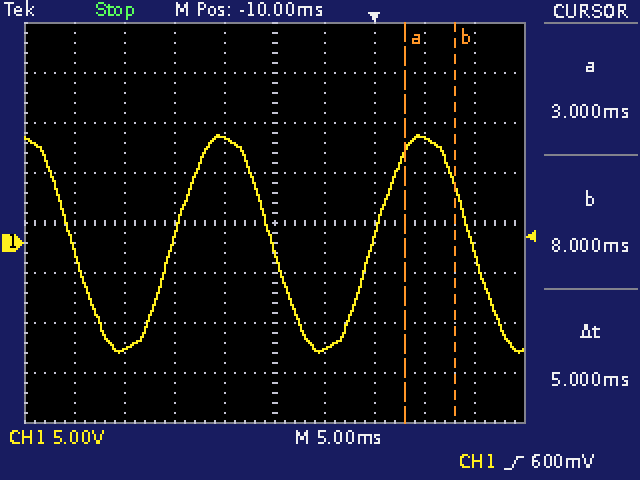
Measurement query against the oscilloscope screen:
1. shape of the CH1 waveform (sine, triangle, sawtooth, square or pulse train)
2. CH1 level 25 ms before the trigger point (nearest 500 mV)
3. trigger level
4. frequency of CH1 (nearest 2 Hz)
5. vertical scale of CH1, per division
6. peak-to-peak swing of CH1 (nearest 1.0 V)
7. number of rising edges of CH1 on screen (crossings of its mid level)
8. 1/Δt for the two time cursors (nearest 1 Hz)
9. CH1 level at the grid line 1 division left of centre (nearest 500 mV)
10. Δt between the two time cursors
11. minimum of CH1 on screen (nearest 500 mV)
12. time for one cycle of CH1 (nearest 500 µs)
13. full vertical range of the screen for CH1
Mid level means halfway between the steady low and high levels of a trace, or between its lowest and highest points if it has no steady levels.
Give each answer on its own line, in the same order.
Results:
sine
-10.5 V
600 mV
50 Hz
5 V
22.0 V
2
200 Hz
10.5 V
5 ms
-11.0 V
20.0 ms
40 V
